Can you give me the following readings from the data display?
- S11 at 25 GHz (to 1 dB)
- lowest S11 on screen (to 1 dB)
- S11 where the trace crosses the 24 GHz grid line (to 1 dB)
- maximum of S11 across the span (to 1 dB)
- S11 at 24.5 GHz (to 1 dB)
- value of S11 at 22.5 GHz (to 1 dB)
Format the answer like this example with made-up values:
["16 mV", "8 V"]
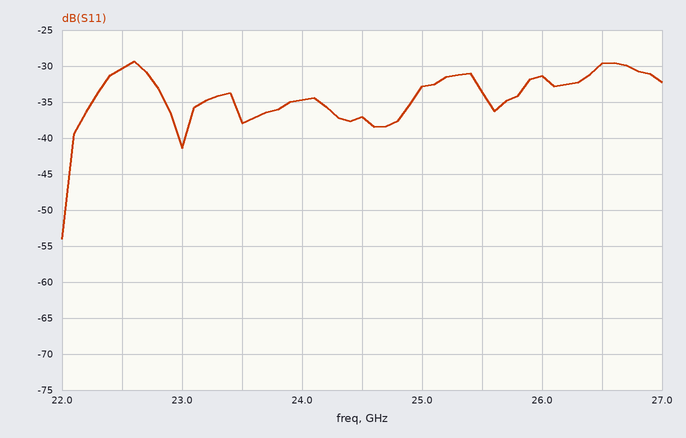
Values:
["-33 dB", "-54 dB", "-35 dB", "-29 dB", "-37 dB", "-30 dB"]
